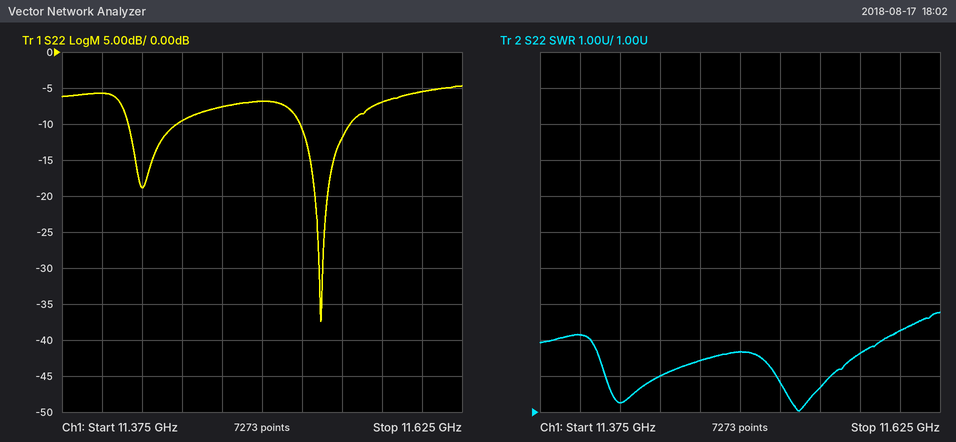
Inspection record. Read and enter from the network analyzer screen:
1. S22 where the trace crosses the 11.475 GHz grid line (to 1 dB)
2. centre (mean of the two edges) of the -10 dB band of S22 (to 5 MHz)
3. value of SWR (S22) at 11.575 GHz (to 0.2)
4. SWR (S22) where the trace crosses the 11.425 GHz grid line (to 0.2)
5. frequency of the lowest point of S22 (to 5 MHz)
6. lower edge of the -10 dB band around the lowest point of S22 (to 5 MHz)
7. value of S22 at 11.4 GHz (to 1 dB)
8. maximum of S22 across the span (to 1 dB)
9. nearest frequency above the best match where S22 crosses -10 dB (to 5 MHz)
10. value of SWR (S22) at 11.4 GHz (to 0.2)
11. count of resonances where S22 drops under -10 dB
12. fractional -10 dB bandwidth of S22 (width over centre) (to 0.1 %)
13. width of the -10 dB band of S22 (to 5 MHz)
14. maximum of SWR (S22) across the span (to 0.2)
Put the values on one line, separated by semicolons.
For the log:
-8 dB; 11.540 GHz; 2.6; 1.2; 11.535 GHz; 11.525 GHz; -6 dB; -5 dB; 11.555 GHz; 3.2; 2; 0.3 %; 30 MHz; 3.8
